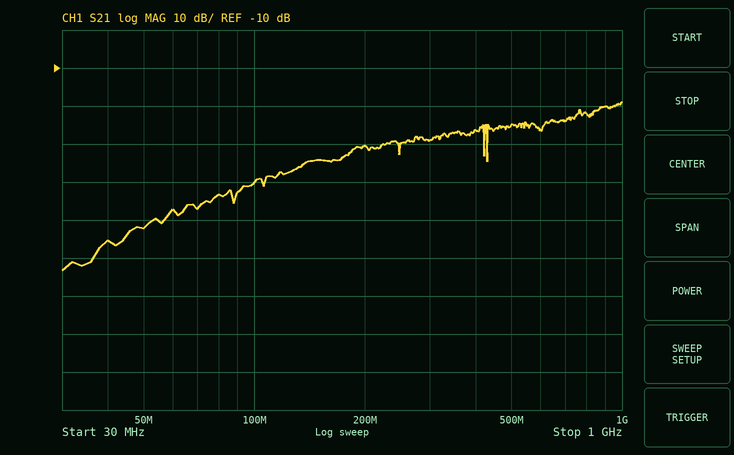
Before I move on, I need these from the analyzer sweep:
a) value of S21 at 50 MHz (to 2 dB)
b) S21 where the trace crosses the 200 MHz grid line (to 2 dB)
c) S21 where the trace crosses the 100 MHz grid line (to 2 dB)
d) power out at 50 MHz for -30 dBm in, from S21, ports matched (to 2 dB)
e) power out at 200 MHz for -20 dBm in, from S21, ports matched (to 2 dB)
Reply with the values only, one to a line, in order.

-52 dB
-30 dB
-40 dB
-82 dBm
-50 dBm
